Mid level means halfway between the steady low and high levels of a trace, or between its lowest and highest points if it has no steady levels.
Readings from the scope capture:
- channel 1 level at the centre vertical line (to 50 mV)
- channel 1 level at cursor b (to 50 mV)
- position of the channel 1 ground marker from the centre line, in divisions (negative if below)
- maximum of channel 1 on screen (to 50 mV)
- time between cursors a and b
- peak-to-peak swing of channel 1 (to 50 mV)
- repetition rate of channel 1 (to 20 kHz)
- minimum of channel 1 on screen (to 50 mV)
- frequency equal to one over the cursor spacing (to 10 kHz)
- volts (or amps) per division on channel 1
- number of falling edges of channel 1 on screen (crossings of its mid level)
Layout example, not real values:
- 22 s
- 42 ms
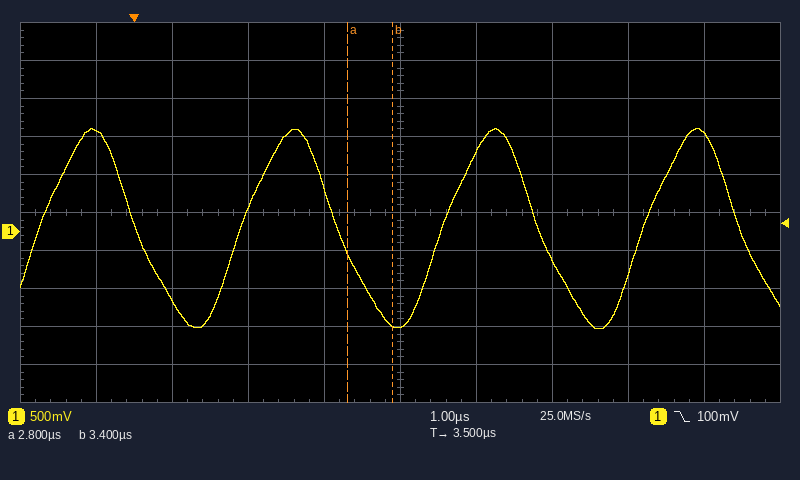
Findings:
- -1.25 V
- -1.25 V
- -0.5 div
- 1.35 V
- 600 ns
- 2.65 V
- 380 kHz
- -1.30 V
- 1.67 MHz
- 500 mV
- 4
